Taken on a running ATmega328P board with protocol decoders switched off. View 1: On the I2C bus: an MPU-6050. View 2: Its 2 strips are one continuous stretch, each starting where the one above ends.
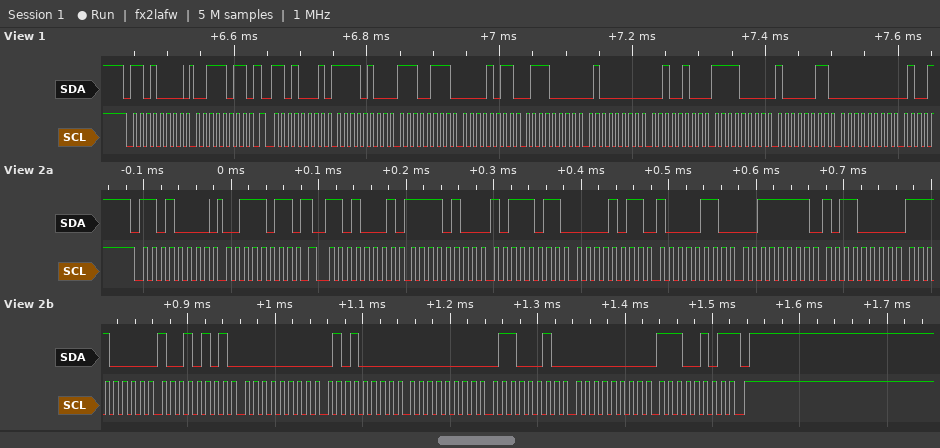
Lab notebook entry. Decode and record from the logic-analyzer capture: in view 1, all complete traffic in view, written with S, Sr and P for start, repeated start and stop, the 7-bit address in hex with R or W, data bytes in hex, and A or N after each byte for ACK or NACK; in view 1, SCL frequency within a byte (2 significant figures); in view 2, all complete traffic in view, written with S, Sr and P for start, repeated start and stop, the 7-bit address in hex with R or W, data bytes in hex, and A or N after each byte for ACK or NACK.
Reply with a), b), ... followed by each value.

a) S 68W A 3B A Sr 68R A F4 A E7 A 0B A 70 A 40 A 24 A F0 A 83 A 00 A
b) 100 kHz
c) S 68W A 3B A Sr 68R A F4 A BB A 0B A 86 A 3F A B0 A F0 A 95 A 00 A 50 A 00 A 62 A 00 A E5 N P
